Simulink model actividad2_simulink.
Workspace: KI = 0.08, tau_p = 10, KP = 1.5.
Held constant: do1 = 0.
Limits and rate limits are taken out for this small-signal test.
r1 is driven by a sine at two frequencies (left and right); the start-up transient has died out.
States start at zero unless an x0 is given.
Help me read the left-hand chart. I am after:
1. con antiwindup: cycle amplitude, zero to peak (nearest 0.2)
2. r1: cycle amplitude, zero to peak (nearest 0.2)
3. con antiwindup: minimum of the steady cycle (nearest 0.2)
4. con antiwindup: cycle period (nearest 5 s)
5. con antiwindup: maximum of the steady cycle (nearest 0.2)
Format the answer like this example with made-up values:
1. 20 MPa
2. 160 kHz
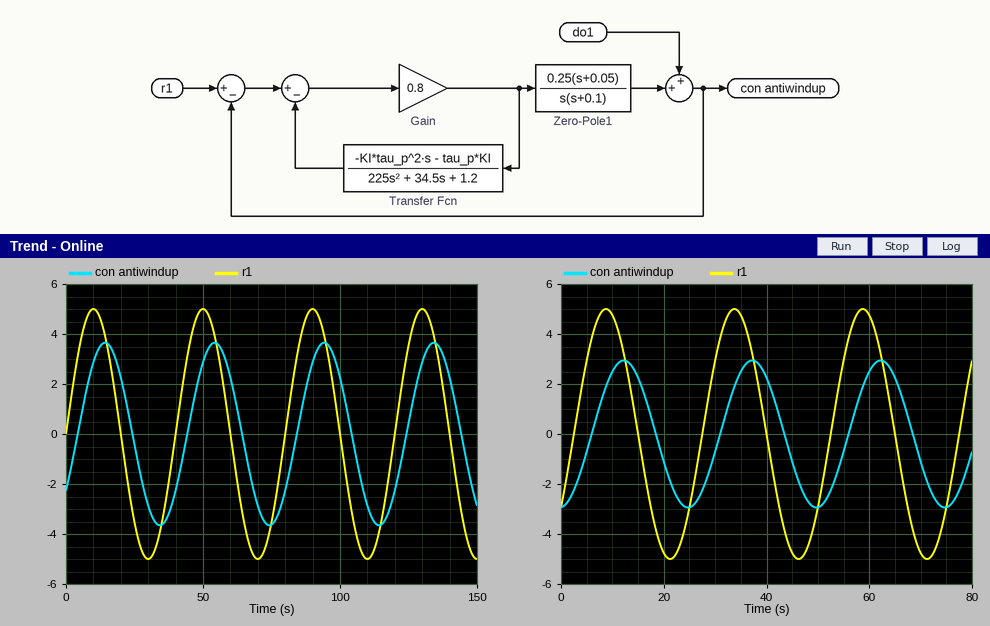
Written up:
1. 3.6
2. 5.0
3. -3.6
4. 40 s
5. 3.6
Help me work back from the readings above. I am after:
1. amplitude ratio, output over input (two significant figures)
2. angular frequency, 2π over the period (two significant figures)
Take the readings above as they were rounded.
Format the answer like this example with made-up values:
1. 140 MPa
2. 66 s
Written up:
1. 0.72
2. 0.16 rad/s
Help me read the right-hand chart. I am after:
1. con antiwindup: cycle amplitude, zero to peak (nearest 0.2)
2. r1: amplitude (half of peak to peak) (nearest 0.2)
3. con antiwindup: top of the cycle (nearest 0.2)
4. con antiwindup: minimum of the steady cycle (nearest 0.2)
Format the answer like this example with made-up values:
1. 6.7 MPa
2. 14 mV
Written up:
1. 3.0
2. 5.0
3. 3.0
4. -3.0
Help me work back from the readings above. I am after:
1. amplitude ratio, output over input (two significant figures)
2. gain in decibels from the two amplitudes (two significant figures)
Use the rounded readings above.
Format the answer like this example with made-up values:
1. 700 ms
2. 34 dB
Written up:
1. 0.60
2. -4.4 dB
